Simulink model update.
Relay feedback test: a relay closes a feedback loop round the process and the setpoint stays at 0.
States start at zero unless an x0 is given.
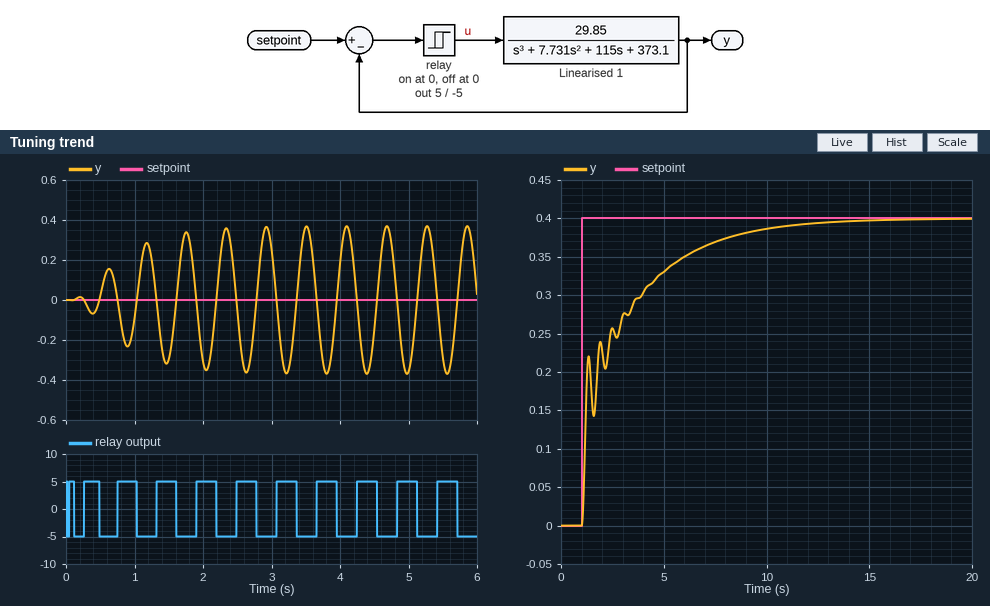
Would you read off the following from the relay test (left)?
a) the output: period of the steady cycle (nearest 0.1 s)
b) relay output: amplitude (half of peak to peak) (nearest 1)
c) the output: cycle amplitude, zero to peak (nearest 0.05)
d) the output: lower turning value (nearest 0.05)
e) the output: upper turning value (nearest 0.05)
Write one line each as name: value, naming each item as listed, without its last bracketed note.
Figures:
the output: period of the steady cycle: 0.6 s
relay output: amplitude (half of peak to peak): 5
the output: cycle amplitude, zero to peak: 0.35
the output: lower turning value: -0.35
the output: upper turning value: 0.35
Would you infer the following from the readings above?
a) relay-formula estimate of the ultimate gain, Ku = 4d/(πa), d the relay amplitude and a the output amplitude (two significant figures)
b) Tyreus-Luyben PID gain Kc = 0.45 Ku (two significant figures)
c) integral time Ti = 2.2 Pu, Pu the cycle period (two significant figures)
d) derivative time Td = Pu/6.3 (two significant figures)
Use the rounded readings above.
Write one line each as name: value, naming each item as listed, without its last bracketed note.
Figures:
relay-formula estimate of the ultimate gain, Ku = 4d/(πa), d the relay amplitude and a the output amplitude: 18
Tyreus-Luyben PID gain Kc = 0.45 Ku: 8.1
integral time Ti = 2.2 Pu, Pu the cycle period: 1.3 s
derivative time Td = Pu/6.3: 0.095 s
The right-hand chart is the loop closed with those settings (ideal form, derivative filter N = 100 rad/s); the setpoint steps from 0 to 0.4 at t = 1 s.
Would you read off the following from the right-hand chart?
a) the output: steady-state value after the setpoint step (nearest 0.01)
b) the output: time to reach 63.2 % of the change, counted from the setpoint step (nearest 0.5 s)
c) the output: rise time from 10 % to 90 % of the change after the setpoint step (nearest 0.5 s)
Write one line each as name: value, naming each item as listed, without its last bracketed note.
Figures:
the output: steady-state value after the setpoint step: 0.40
the output: time to reach 63.2 % of the change, counted from the setpoint step: 1.5 s
the output: rise time from 10 % to 90 % of the change after the setpoint step: 5.5 s
